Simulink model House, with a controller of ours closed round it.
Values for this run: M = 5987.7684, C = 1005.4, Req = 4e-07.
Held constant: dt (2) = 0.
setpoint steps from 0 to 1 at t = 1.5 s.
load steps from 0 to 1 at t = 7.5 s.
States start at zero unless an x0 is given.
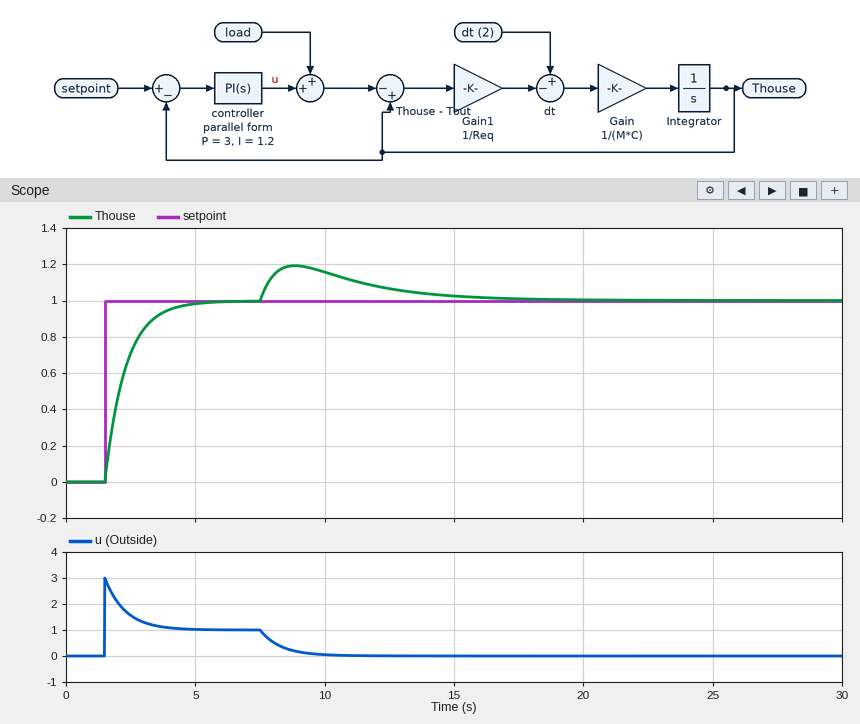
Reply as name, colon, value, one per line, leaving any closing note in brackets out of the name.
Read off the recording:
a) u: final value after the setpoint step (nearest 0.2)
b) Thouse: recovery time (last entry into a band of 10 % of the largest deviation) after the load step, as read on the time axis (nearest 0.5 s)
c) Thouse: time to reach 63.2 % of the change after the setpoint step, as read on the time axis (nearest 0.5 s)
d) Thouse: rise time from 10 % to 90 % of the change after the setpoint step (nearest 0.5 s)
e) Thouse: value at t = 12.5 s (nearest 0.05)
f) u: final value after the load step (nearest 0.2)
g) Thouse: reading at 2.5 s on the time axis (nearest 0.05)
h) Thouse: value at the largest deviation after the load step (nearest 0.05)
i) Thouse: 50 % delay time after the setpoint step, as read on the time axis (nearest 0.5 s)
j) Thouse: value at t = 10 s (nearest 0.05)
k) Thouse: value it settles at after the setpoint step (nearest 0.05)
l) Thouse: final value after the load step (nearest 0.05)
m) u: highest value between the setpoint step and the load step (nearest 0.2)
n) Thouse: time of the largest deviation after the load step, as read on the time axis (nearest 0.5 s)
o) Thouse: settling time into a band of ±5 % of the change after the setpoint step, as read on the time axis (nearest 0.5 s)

u: final value after the setpoint step: 1.0
Thouse: recovery time (last entry into a band of 10 % of the largest deviation) after the load step, as read on the time axis: 15.5 s
Thouse: time to reach 63.2 % of the change after the setpoint step, as read on the time axis: 2.5 s
Thouse: rise time from 10 % to 90 % of the change after the setpoint step: 2.0 s
Thouse: value at t = 12.5 s: 1.05
u: final value after the load step: 0.0
Thouse: reading at 2.5 s on the time axis: 0.70
Thouse: value at the largest deviation after the load step: 1.20
Thouse: 50 % delay time after the setpoint step, as read on the time axis: 2.0 s
Thouse: value at t = 10 s: 1.15
Thouse: value it settles at after the setpoint step: 1.00
Thouse: final value after the load step: 1.00
u: highest value between the setpoint step and the load step: 3.0
Thouse: time of the largest deviation after the load step, as read on the time axis: 9.0 s
Thouse: settling time into a band of ±5 % of the change after the setpoint step, as read on the time axis: 4.0 s
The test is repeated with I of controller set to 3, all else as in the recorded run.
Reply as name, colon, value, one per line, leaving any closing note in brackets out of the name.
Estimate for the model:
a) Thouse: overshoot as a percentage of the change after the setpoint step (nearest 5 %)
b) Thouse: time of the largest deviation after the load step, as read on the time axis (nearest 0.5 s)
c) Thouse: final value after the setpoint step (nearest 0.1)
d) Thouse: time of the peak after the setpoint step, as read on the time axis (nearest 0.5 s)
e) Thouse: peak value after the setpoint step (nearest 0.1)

Thouse: overshoot as a percentage of the change after the setpoint step: 10 %
Thouse: time of the largest deviation after the load step, as read on the time axis: 8.5 s
Thouse: final value after the setpoint step: 1.0
Thouse: time of the peak after the setpoint step, as read on the time axis: 4.0 s
Thouse: peak value after the setpoint step: 1.1
